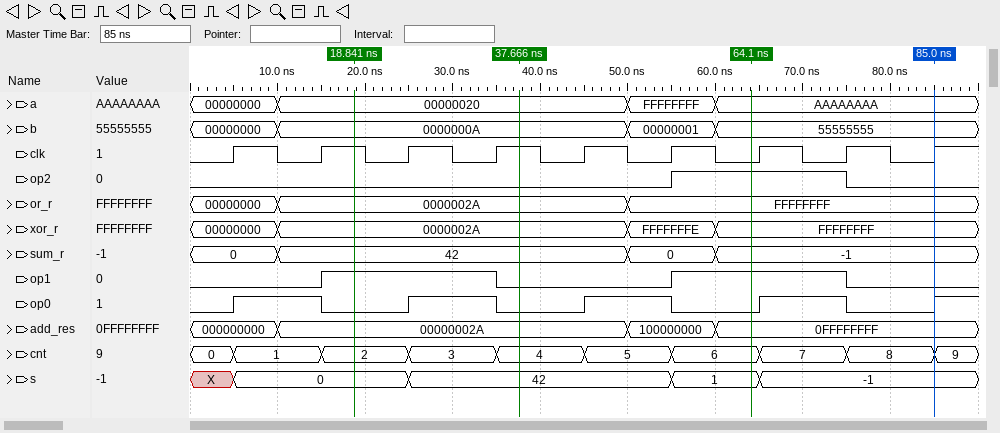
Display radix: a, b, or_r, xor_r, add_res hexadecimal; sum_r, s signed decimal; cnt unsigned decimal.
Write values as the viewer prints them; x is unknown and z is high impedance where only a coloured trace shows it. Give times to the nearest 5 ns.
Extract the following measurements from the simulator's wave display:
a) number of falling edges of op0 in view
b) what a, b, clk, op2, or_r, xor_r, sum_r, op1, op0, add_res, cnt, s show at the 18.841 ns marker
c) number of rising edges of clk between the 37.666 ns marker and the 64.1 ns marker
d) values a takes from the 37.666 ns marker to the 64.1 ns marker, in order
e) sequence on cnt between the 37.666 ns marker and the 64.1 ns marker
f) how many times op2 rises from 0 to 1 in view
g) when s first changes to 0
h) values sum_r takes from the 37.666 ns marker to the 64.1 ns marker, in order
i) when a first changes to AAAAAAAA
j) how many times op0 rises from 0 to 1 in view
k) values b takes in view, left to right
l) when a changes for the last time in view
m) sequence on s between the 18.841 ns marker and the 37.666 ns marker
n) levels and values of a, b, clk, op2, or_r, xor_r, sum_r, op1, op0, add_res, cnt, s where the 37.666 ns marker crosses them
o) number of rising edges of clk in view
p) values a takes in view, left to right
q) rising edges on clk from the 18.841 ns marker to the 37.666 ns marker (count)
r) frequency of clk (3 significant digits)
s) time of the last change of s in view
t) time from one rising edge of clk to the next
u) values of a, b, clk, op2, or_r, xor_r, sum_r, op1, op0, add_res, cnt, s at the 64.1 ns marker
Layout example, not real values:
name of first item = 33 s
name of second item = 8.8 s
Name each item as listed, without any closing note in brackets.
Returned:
number of falling edges of op0 in view = 4
what a, b, clk, op2, or_r, xor_r, sum_r, op1, op0, add_res, cnt, s show at the 18.841 ns marker = a=00000020, b=0000000A, clk=1, op2=0, or_r=0000002A, xor_r=0000002A, sum_r=42, op1=1, op0=0, add_res=00000002A, cnt=2, s=0
number of rising edges of clk between the 37.666 ns marker and the 64.1 ns marker = 2
values a takes from the 37.666 ns marker to the 64.1 ns marker, in order = 00000020, FFFFFFFF, AAAAAAAA
sequence on cnt between the 37.666 ns marker and the 64.1 ns marker = 4, 5, 6
how many times op2 rises from 0 to 1 in view = 1
when s first changes to 0 = 5 ns
values sum_r takes from the 37.666 ns marker to the 64.1 ns marker, in order = 42, 0, -1
when a first changes to AAAAAAAA = 60 ns
how many times op0 rises from 0 to 1 in view = 5
values b takes in view, left to right = 00000000, 0000000A, 00000001, 55555555
when a changes for the last time in view = 60 ns
sequence on s between the 18.841 ns marker and the 37.666 ns marker = 0, 42
levels and values of a, b, clk, op2, or_r, xor_r, sum_r, op1, op0, add_res, cnt, s where the 37.666 ns marker crosses them = a=00000020, b=0000000A, clk=1, op2=0, or_r=0000002A, xor_r=0000002A, sum_r=42, op1=0, op0=0, add_res=00000002A, cnt=4, s=42
number of rising edges of clk in view = 9
values a takes in view, left to right = 00000000, 00000020, FFFFFFFF, AAAAAAAA
rising edges on clk from the 18.841 ns marker to the 37.666 ns marker = 2
frequency of clk = 100 MHz
time of the last change of s in view = 65 ns
time from one rising edge of clk to the next = 10 ns
values of a, b, clk, op2, or_r, xor_r, sum_r, op1, op0, add_res, cnt, s at the 64.1 ns marker = a=AAAAAAAA, b=55555555, clk=0, op2=1, or_r=FFFFFFFF, xor_r=FFFFFFFF, sum_r=-1, op1=1, op0=0, add_res=0FFFFFFFF, cnt=6, s=1
